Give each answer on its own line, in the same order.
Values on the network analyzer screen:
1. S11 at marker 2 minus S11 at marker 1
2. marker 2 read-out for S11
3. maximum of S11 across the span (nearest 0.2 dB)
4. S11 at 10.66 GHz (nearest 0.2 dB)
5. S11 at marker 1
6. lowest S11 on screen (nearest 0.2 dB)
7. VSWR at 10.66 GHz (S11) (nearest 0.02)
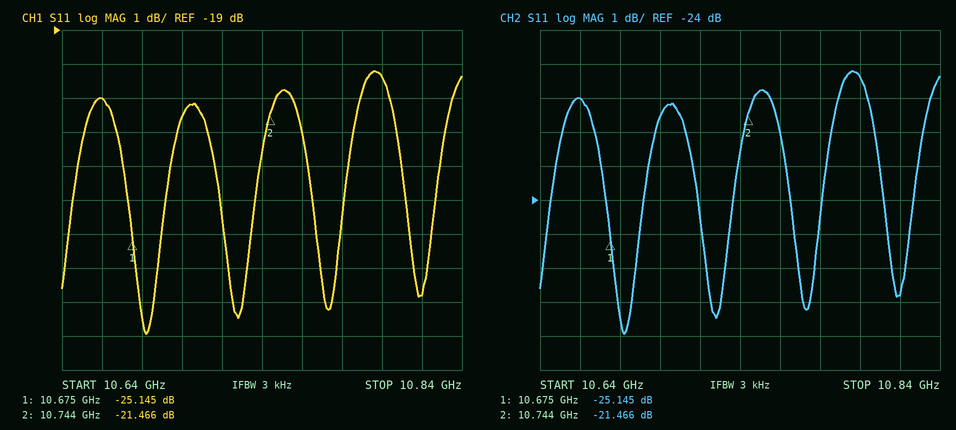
3.679 dB
-21.466 dB
-20.2 dB
-21.0 dB
-25.145 dB
-28.0 dB
1.20
